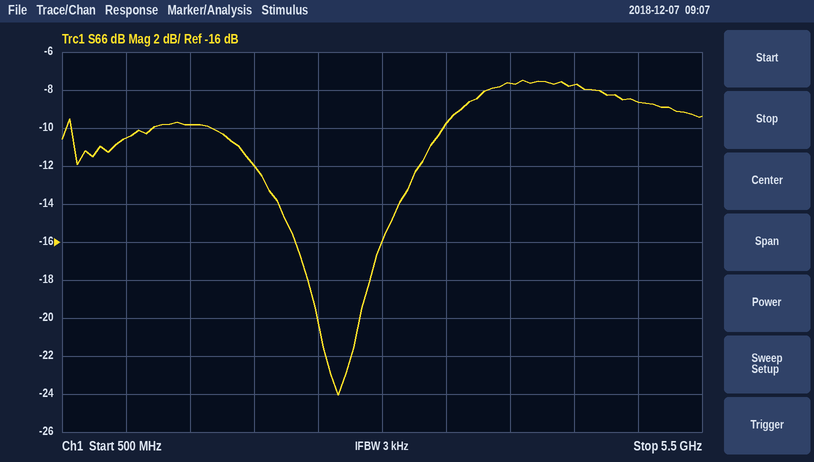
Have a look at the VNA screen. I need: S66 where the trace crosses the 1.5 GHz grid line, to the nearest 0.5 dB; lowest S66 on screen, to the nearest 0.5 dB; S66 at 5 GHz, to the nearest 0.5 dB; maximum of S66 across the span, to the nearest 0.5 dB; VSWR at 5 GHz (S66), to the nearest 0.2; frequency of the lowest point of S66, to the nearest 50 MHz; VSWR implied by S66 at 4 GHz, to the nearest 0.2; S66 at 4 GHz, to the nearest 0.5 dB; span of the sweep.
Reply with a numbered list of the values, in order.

1. -10.0 dB
2. -24.0 dB
3. -8.5 dB
4. -7.5 dB
5. 2.2
6. 2.65 GHz
7. 2.4
8. -7.5 dB
9. 5 GHz
